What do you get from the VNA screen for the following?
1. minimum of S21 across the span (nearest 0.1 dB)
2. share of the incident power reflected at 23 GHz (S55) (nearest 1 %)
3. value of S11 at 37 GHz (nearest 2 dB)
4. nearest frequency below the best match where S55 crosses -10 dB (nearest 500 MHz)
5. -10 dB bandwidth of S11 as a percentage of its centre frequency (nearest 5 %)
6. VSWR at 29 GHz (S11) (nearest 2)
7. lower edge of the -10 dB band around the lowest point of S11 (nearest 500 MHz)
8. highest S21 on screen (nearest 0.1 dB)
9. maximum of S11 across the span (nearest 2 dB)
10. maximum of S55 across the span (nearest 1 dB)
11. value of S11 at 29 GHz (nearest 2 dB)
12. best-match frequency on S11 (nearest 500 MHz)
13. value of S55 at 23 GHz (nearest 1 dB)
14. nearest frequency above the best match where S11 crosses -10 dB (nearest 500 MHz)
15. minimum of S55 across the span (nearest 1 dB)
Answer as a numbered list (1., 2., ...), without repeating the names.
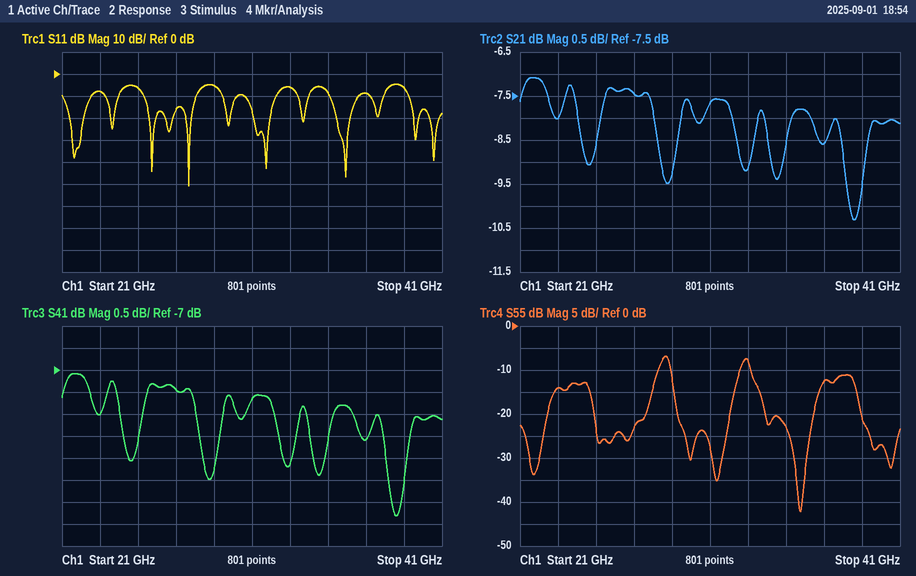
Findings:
1. -10.3 dB
2. 4 %
3. -8 dB
4. 33.0 GHz
5. 10 %
6. 4
7. 25.5 GHz
8. -7.1 dB
9. -4 dB
10. -7 dB
11. -6 dB
12. 27.5 GHz
13. -14 dB
14. 28.0 GHz
15. -42 dB
